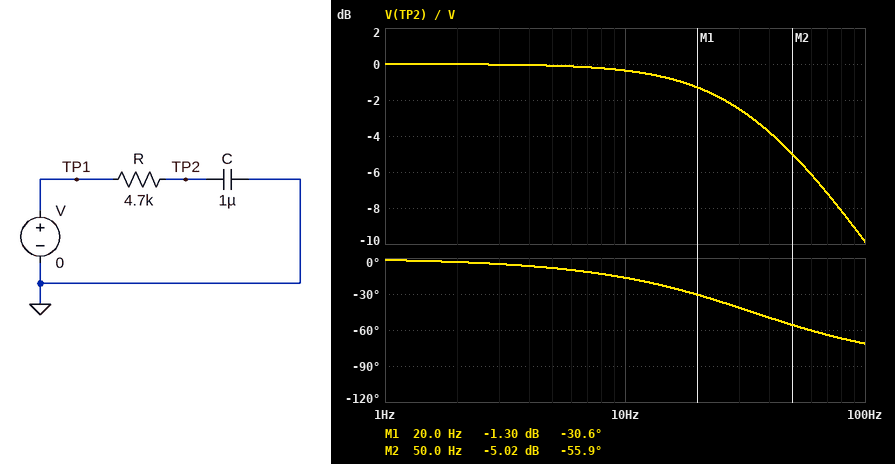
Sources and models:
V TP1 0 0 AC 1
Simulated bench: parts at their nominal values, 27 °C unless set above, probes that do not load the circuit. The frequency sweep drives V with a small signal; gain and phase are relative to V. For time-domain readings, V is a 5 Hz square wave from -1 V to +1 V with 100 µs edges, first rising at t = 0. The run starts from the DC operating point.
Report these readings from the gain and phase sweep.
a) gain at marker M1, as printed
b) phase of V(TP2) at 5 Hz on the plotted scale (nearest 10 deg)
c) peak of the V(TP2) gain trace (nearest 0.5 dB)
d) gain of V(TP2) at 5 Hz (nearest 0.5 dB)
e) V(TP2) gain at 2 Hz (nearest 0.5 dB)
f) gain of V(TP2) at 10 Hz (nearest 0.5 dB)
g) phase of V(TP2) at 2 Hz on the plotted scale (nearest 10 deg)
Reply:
-1.30 dB
-10 deg
0 dB
0 dB
0 dB
-0.5 dB
0 deg
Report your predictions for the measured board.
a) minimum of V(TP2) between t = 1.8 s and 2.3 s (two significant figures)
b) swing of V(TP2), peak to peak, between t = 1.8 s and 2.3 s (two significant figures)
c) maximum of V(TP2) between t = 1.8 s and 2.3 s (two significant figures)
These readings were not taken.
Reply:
-1.0 V
2.0 V
1.0 V
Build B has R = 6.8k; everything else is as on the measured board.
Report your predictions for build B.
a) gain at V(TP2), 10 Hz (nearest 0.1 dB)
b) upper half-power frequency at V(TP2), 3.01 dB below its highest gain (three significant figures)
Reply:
-0.7 dB
23.4 Hz
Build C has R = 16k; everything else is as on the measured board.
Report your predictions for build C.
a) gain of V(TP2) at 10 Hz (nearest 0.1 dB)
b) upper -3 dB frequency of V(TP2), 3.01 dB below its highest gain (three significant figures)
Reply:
-3.0 dB
9.95 Hz
